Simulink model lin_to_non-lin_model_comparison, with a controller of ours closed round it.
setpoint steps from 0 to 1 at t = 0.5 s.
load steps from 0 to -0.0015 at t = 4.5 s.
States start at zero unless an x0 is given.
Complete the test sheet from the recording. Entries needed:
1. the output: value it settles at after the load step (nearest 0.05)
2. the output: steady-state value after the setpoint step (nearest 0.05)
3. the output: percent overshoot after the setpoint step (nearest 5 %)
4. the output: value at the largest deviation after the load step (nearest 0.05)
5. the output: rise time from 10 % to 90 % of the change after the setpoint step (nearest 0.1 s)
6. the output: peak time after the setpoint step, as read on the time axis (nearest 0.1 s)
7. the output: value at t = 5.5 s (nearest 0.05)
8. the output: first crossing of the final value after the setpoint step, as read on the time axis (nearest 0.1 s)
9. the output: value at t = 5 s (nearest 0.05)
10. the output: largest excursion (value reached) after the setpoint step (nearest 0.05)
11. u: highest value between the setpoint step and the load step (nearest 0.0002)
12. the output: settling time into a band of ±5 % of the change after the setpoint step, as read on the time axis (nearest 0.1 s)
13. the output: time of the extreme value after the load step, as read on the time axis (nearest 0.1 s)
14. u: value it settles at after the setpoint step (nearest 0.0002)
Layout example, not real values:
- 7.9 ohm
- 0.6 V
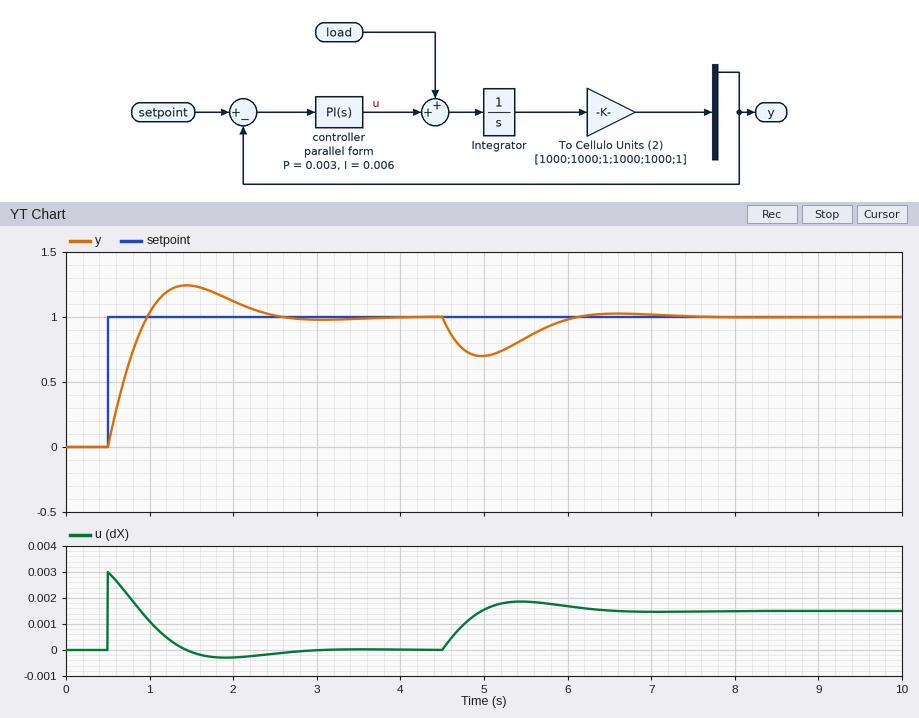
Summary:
- 1.00
- 1.00
- 25 %
- 0.70
- 0.4 s
- 1.4 s
- 0.85
- 1.0 s
- 0.70
- 1.25
- 0.0030
- 2.3 s
- 5.0 s
- 0.0000
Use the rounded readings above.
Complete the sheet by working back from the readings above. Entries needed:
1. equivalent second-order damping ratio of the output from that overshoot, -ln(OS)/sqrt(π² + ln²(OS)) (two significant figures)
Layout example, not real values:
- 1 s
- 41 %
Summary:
- 0.40
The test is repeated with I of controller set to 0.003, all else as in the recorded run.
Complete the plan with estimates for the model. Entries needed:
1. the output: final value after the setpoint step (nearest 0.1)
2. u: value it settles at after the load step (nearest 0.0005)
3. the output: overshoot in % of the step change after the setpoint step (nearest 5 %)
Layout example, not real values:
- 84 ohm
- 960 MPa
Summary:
- 1.0
- 0.0015
- 15 %
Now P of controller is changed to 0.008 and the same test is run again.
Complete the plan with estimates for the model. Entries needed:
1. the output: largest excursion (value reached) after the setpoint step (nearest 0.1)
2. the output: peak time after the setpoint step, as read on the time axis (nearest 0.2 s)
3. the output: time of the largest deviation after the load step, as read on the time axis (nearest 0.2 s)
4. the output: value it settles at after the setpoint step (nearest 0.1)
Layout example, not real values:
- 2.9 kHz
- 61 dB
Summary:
- 1.1
- 1.2 s
- 4.8 s
- 1.0
